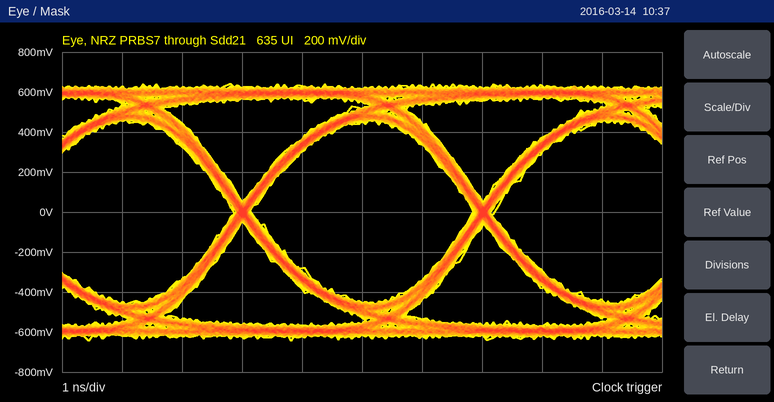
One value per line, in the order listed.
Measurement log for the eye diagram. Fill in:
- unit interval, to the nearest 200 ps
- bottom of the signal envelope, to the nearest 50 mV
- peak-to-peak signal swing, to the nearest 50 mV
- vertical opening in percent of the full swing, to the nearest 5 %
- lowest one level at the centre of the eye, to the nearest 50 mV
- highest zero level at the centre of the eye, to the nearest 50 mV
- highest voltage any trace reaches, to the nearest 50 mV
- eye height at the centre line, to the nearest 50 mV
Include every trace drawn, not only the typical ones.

4.0 ns
-650 mV
1.30 V
70 %
450 mV
-450 mV
650 mV
900 mV
